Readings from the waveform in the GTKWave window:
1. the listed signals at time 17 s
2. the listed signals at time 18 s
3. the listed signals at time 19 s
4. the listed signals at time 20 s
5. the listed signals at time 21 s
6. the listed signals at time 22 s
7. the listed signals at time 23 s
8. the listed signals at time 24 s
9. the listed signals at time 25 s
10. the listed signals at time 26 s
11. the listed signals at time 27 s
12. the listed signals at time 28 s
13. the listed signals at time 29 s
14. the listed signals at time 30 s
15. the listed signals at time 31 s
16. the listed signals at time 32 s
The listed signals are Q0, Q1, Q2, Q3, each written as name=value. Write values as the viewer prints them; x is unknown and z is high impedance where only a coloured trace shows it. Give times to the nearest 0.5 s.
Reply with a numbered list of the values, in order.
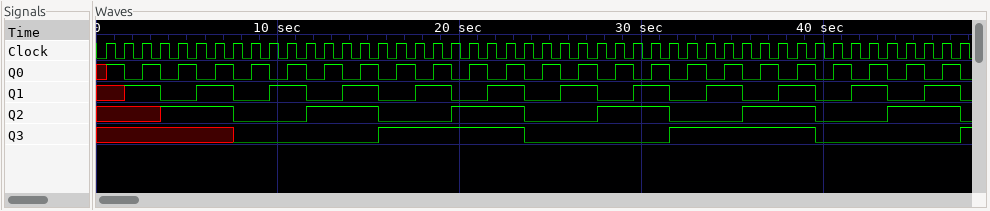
1. Q0=1, Q1=0, Q2=0, Q3=1
2. Q0=0, Q1=1, Q2=0, Q3=1
3. Q0=1, Q1=1, Q2=0, Q3=1
4. Q0=0, Q1=0, Q2=1, Q3=1
5. Q0=1, Q1=0, Q2=1, Q3=1
6. Q0=0, Q1=1, Q2=1, Q3=1
7. Q0=1, Q1=1, Q2=1, Q3=1
8. Q0=0, Q1=0, Q2=0, Q3=0
9. Q0=1, Q1=0, Q2=0, Q3=0
10. Q0=0, Q1=1, Q2=0, Q3=0
11. Q0=1, Q1=1, Q2=0, Q3=0
12. Q0=0, Q1=0, Q2=1, Q3=0
13. Q0=1, Q1=0, Q2=1, Q3=0
14. Q0=0, Q1=1, Q2=1, Q3=0
15. Q0=1, Q1=1, Q2=1, Q3=0
16. Q0=0, Q1=0, Q2=0, Q3=1
